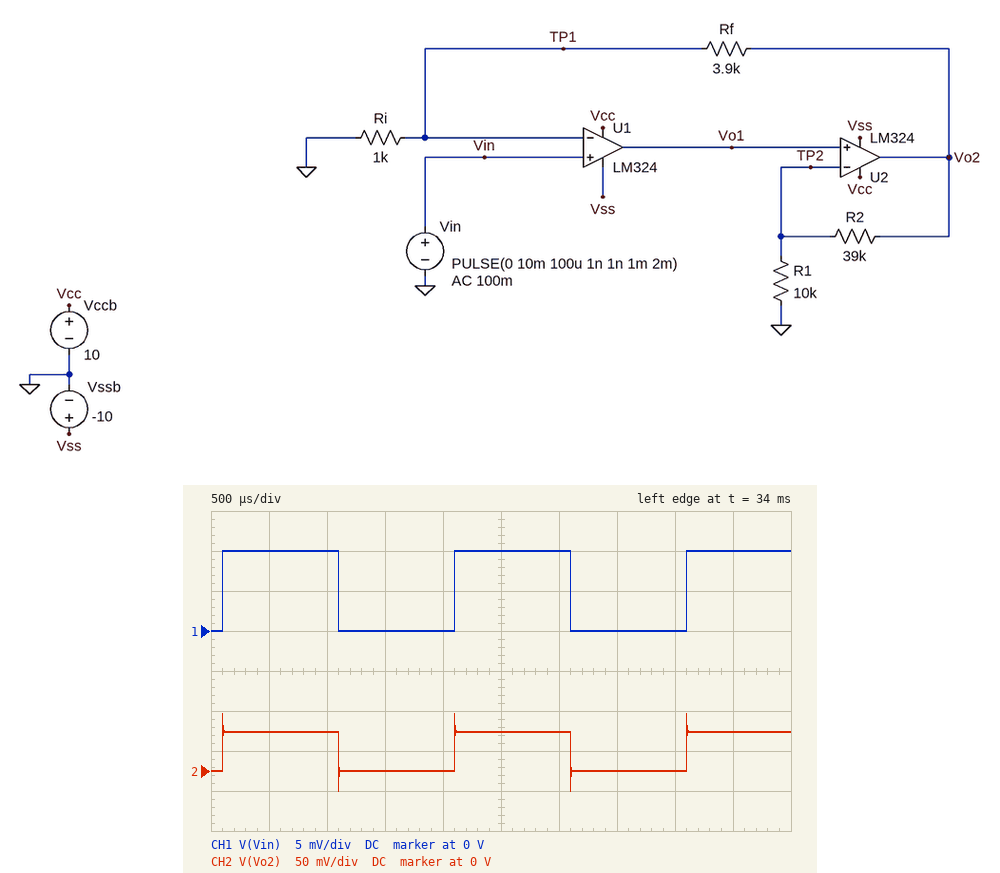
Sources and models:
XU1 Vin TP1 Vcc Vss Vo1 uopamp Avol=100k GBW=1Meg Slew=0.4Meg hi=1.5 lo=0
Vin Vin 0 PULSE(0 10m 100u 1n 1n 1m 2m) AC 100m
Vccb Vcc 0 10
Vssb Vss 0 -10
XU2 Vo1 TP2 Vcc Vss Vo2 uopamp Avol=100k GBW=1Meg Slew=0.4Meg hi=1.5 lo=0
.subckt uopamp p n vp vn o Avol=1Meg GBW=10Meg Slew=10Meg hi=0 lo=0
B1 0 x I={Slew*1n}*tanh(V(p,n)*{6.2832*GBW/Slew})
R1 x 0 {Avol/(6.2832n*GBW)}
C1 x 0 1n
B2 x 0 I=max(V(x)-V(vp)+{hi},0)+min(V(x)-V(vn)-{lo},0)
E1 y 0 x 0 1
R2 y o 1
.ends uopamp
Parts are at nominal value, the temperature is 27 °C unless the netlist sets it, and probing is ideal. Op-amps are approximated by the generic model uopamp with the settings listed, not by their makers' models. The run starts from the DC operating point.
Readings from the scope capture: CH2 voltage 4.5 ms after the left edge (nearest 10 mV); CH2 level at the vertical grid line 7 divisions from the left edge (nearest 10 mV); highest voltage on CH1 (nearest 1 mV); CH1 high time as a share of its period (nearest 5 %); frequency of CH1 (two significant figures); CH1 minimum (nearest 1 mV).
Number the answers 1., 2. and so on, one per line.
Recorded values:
1. 50 mV
2. 0 V
3. 10 mV
4. 50 %
5. 500 Hz
6. 0 V
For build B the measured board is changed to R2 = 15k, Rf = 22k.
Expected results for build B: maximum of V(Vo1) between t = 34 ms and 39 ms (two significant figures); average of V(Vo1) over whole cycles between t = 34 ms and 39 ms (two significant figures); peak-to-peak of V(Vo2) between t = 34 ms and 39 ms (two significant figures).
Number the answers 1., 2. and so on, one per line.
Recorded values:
1. 92 mV
2. 46 mV
3. 230 mV
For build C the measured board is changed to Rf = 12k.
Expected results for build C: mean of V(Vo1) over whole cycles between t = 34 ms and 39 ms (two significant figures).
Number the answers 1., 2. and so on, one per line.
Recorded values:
1. 13 mV
